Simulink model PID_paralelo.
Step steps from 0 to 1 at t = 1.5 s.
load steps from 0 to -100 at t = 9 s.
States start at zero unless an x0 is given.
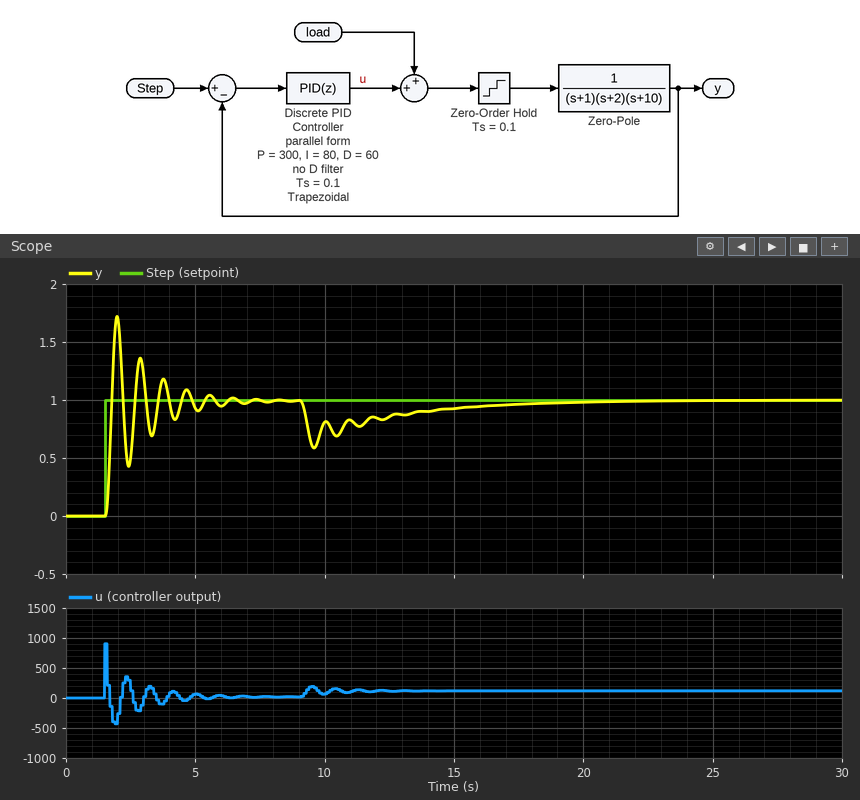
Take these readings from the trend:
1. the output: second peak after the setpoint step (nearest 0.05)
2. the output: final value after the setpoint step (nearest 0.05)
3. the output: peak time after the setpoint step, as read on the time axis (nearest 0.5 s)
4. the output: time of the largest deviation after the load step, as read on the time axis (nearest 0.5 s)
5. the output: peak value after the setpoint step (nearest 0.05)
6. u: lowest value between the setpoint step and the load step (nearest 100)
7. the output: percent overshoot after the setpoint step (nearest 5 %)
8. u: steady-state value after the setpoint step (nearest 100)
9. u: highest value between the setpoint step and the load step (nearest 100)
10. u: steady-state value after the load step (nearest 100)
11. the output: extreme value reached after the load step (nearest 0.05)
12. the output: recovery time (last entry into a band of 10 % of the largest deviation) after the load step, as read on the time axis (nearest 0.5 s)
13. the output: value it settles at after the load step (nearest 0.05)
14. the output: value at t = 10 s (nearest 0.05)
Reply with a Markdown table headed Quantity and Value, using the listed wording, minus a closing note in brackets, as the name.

| Quantity | Value |
|---|---|
| the output: second peak after the setpoint step | 1.35 |
| the output: final value after the setpoint step | 1.00 |
| the output: peak time after the setpoint step, as read on the time axis | 2.0 s |
| the output: time of the largest deviation after the load step, as read on the time axis | 9.5 s |
| the output: peak value after the setpoint step | 1.70 |
| u: lowest value between the setpoint step and the load step | -400 |
| the output: percent overshoot after the setpoint step | 70 % |
| u: steady-state value after the setpoint step | 0 |
| u: highest value between the setpoint step and the load step | 900 |
| u: steady-state value after the load step | 100 |
| the output: extreme value reached after the load step | 0.60 |
| the output: recovery time (last entry into a band of 10 % of the largest deviation) after the load step, as read on the time axis | 17.0 s |
| the output: value it settles at after the load step | 1.00 |
| the output: value at t = 10 s | 0.80 |
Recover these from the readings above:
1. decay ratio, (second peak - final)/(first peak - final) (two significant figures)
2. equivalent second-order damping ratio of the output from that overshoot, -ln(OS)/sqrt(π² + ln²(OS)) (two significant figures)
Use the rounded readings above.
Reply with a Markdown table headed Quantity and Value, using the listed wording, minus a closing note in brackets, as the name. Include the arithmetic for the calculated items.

| Quantity | Value |
|---|---|
| decay ratio, (second peak - final)/(first peak - final) | (1.35 - 1) / (1.7 - 1) = 0.50 |
| equivalent second-order damping ratio of the output from that overshoot, -ln(OS)/sqrt(π² + ln²(OS)) | ln(0.7) = -0.357; 0.357 / sqrt(9.870 + 0.127) = 0.11 |
